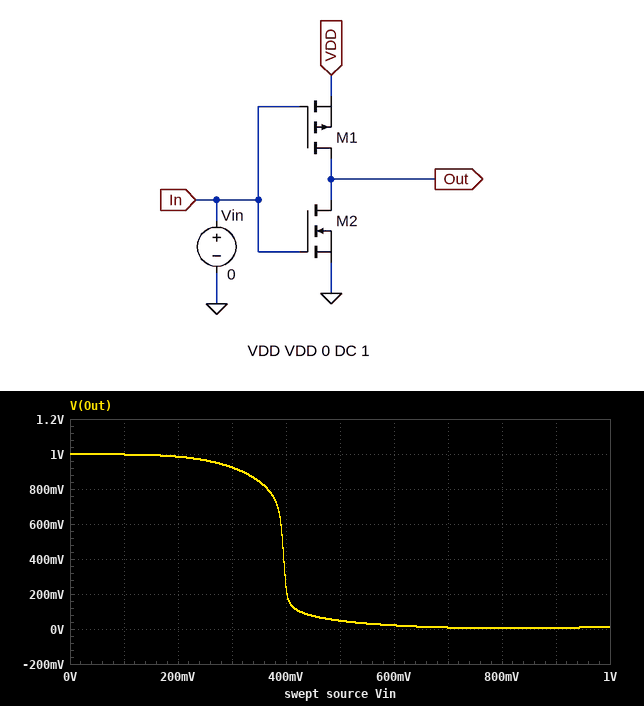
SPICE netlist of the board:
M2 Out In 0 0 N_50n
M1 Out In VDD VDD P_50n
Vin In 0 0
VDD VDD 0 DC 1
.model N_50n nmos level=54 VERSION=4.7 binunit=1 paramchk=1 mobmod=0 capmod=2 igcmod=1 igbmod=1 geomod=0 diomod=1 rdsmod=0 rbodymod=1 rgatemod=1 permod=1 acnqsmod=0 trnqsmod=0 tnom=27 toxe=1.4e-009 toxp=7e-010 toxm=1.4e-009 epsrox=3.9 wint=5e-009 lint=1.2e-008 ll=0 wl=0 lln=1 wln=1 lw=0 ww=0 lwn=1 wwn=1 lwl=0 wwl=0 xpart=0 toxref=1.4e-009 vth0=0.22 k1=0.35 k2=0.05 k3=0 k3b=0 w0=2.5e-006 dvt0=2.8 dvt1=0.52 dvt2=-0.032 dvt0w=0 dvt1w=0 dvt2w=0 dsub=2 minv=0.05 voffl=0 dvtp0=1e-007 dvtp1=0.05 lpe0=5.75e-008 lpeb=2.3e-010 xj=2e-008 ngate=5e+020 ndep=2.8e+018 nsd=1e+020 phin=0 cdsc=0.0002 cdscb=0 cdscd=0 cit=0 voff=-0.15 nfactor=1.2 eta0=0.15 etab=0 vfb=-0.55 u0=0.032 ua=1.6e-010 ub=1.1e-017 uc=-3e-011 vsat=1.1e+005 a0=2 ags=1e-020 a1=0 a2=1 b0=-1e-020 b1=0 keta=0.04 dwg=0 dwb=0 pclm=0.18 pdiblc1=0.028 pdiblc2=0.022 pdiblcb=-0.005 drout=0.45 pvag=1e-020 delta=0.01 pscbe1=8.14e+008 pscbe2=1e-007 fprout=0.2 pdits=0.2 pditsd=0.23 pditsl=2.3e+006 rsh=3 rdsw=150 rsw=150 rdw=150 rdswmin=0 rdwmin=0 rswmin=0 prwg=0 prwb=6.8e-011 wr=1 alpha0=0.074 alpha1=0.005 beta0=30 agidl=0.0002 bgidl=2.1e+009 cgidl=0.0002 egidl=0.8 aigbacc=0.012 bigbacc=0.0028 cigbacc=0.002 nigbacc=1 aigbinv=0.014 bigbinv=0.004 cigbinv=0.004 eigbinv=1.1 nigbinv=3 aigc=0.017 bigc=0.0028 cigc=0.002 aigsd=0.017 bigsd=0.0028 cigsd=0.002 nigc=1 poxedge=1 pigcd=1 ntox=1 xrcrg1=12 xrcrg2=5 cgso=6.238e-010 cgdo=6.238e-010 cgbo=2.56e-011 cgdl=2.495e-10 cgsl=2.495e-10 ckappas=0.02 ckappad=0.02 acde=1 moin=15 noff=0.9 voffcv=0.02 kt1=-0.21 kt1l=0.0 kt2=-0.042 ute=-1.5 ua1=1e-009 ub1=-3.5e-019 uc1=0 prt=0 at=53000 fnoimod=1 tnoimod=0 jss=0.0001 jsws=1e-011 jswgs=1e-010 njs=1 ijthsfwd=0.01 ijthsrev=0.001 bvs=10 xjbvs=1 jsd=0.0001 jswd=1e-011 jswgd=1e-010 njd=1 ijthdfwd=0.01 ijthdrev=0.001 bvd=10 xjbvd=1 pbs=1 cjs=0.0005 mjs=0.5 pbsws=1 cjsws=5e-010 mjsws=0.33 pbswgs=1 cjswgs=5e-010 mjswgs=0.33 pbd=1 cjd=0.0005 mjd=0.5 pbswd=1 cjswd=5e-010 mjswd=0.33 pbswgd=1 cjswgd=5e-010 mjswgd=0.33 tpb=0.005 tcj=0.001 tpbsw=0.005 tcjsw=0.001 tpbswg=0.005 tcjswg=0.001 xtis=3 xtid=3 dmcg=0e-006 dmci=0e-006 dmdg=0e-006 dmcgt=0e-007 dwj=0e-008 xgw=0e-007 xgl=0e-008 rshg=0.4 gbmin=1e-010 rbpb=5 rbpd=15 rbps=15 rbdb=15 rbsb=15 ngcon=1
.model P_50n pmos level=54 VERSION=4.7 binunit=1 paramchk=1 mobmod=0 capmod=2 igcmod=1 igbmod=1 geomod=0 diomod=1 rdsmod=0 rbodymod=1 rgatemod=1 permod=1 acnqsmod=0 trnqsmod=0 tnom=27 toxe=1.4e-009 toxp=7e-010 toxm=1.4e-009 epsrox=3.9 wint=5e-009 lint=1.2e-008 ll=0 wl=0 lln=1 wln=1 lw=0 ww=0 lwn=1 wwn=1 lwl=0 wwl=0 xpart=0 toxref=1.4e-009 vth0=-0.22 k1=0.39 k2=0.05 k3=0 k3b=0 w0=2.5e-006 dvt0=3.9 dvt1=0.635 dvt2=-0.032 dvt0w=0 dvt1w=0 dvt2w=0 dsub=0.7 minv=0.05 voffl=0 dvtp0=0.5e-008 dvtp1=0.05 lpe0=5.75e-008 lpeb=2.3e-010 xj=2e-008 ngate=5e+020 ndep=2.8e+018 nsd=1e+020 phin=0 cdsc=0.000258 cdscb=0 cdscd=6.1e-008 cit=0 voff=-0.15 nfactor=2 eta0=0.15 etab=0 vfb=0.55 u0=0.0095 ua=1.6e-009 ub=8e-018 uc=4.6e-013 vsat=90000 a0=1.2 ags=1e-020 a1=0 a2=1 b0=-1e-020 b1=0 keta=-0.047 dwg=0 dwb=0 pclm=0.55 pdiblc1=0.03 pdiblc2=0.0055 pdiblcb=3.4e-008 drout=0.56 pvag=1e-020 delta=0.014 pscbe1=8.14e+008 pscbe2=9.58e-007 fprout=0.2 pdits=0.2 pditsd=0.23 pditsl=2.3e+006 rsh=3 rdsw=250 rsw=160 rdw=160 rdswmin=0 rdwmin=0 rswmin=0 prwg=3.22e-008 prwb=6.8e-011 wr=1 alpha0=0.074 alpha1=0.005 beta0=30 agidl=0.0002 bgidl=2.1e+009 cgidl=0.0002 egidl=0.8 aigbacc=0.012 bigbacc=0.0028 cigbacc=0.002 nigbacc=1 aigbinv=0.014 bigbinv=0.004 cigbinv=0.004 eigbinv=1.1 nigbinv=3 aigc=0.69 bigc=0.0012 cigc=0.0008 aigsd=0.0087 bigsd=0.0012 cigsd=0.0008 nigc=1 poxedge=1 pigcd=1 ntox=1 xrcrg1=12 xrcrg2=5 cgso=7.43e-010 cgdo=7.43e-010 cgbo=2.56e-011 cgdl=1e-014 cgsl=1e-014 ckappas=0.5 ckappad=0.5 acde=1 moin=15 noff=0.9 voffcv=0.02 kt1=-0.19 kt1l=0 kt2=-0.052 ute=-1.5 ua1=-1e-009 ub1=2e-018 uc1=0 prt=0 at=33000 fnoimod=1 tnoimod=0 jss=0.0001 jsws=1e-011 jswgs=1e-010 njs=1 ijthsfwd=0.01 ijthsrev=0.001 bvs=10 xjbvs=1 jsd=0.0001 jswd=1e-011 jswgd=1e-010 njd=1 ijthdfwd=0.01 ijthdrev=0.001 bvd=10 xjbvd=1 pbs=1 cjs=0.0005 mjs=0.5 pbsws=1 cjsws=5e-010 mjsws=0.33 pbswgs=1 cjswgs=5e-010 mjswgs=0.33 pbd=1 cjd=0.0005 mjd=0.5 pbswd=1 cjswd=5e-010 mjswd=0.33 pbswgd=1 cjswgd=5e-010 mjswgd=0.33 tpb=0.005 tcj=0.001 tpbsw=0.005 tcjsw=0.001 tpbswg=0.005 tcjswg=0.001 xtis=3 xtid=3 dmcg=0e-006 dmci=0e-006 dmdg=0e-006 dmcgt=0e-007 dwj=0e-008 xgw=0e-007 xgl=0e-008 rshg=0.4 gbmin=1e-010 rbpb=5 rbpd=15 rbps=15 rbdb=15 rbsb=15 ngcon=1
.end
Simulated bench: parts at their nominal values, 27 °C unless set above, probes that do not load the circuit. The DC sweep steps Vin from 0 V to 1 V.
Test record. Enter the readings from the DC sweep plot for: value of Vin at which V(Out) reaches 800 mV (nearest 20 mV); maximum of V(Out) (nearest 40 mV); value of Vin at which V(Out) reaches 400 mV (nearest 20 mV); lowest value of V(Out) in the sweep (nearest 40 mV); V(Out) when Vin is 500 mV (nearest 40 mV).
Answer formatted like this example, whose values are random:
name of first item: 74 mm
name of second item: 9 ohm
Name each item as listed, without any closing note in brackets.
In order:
value of Vin at which V(Out) reaches 800 mV: 360 mV
maximum of V(Out): 1.00 V
value of Vin at which V(Out) reaches 400 mV: 400 mV
lowest value of V(Out) in the sweep: 0 V
V(Out) when Vin is 500 mV: 40 mV
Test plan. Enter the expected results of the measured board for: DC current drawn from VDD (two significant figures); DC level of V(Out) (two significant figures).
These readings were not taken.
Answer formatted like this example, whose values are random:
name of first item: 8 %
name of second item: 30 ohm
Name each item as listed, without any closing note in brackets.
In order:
DC current drawn from VDD: 980 nA
DC level of V(Out): 1.0 V
